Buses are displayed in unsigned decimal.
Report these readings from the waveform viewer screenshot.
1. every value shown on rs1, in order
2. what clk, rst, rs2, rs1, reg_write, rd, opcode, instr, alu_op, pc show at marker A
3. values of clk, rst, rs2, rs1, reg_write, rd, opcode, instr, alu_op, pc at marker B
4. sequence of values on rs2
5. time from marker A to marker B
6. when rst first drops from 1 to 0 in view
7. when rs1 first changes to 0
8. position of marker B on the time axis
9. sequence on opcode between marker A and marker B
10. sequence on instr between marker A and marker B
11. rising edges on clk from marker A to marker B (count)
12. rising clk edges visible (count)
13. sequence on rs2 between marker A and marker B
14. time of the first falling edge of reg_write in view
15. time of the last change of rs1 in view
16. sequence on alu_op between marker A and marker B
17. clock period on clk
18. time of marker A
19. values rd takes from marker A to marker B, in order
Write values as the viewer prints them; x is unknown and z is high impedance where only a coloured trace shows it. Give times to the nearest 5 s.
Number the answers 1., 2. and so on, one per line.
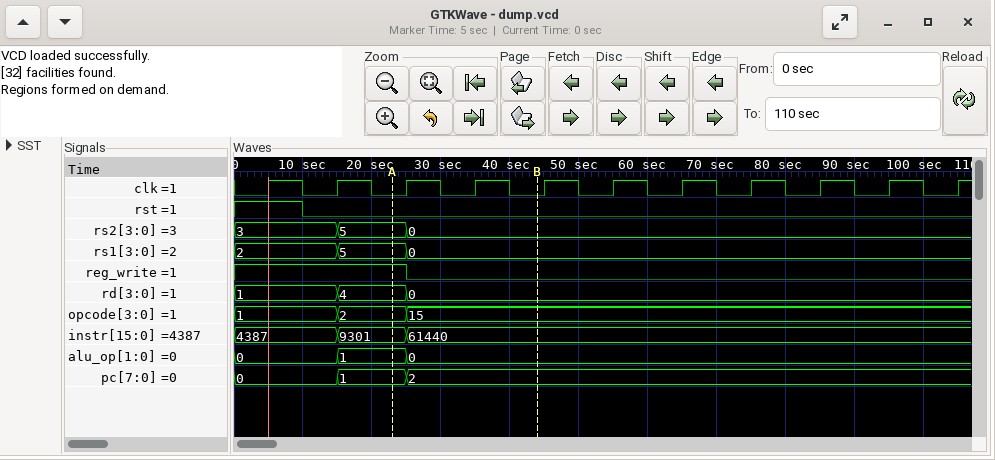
1. 2, 5, 0
2. clk=0, rst=0, rs2=5, rs1=5, reg_write=1, rd=4, opcode=2, instr=9301, alu_op=1, pc=1
3. clk=0, rst=0, rs2=0, rs1=0, reg_write=0, rd=0, opcode=15, instr=61440, alu_op=0, pc=2
4. 3, 5, 0
5. 20 s
6. 10 s
7. 25 s
8. 45 s
9. 2, 15
10. 9301, 61440
11. 2
12. 11
13. 5, 0
14. 25 s
15. 25 s
16. 1, 0
17. 10 s
18. 25 s
19. 4, 0
